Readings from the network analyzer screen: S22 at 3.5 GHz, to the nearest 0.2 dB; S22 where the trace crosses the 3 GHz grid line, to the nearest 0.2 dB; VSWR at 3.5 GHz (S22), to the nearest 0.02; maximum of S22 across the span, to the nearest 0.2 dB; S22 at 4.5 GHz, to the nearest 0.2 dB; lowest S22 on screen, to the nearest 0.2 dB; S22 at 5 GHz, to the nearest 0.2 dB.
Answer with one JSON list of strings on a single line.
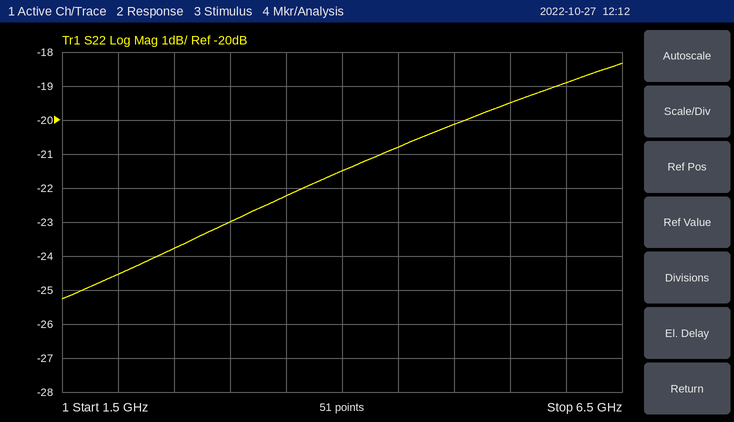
["-22.2 dB", "-23.0 dB", "1.16", "-18.4 dB", "-20.8 dB", "-25.2 dB", "-20.2 dB"]
